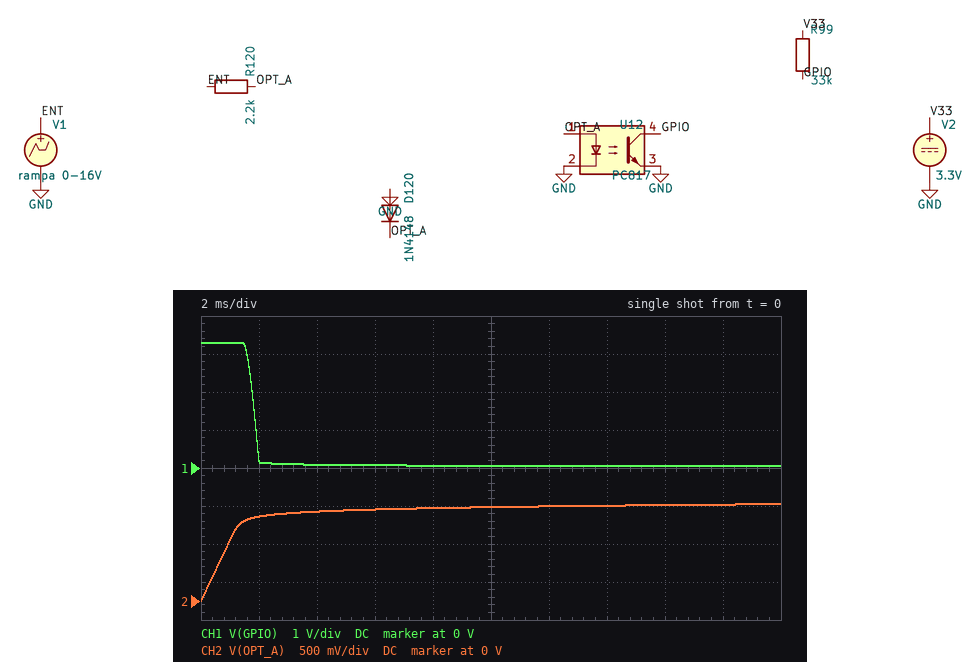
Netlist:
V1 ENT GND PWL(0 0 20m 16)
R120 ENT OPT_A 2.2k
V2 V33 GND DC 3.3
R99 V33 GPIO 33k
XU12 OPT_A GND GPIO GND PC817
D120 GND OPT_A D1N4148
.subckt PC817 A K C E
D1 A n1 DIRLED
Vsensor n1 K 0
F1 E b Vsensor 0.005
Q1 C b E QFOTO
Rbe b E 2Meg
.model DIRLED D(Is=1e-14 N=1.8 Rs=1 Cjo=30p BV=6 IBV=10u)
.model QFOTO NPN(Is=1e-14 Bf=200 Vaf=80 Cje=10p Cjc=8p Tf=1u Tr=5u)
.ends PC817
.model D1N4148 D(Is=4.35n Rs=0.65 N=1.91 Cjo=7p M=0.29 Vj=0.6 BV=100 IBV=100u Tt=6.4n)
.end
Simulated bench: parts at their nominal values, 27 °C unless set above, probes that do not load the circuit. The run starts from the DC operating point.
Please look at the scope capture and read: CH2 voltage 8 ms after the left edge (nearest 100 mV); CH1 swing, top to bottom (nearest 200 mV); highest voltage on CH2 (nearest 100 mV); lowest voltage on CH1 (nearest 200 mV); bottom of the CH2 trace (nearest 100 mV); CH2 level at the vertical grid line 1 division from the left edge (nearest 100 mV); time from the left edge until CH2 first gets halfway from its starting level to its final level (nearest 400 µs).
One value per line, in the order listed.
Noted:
1.2 V
3.2 V
1.3 V
0 V
0 V
1.1 V
800 µs
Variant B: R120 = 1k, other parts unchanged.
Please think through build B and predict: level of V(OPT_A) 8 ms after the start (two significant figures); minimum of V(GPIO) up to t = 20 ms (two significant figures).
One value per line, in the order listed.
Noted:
1.3 V
32 mV
